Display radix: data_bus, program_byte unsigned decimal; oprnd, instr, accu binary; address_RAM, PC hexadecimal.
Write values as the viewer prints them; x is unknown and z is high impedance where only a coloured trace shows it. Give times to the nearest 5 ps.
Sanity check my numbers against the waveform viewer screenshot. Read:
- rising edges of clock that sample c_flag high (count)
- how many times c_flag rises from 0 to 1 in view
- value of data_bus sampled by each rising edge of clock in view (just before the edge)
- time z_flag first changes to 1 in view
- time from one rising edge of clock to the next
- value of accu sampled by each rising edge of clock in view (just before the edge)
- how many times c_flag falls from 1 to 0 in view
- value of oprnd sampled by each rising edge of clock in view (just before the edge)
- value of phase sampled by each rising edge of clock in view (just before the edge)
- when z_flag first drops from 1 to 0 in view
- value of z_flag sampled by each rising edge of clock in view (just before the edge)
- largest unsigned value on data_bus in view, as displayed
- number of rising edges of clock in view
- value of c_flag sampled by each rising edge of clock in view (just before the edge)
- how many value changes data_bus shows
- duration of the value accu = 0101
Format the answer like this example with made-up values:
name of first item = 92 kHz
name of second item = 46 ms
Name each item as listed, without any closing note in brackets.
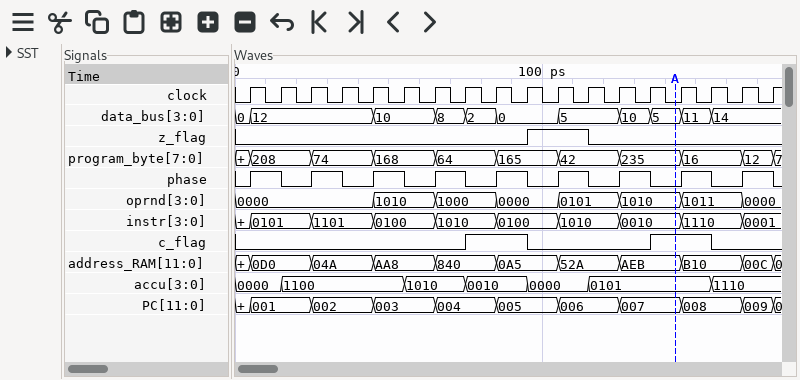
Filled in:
rising edges of clock that sample c_flag high = 4
how many times c_flag rises from 0 to 1 in view = 2
value of data_bus sampled by each rising edge of clock in view = 0, 12, 12, 12, 12, 10, 10, 8, 2, 0, 0, 5, 5, 10, 5, 11, 14, 14
time z_flag first changes to 1 in view = 95 ps
time from one rising edge of clock to the next = 10 ps
value of accu sampled by each rising edge of clock in view = 0000, 0000, 1100, 1100, 1100, 1100, 1010, 1010, 0010, 0010, 0000, 0000, 0101, 0101, 0101, 0101, 1110, 1110
how many times c_flag falls from 1 to 0 in view = 2
value of oprnd sampled by each rising edge of clock in view = 0000, 0000, 0000, 0000, 0000, 1010, 1010, 1000, 1000, 0000, 0000, 0101, 0101, 1010, 1010, 1011, 1011, 0000
value of phase sampled by each rising edge of clock in view = 0 1 0 1 0 1 0 1 0 1 0 1 0 1 0 1 0 1
when z_flag first drops from 1 to 0 in view = 115 ps
value of z_flag sampled by each rising edge of clock in view = 0 0 0 0 0 0 0 0 0 0 1 1 0 0 0 0 0 0
largest unsigned value on data_bus in view, as displayed = 14
number of rising edges of clock in view = 18
value of c_flag sampled by each rising edge of clock in view = 0 0 0 0 0 0 0 0 1 1 0 0 0 0 1 1 0 0
how many value changes data_bus shows = 10
duration of the value accu = 0101 = 40 ps
